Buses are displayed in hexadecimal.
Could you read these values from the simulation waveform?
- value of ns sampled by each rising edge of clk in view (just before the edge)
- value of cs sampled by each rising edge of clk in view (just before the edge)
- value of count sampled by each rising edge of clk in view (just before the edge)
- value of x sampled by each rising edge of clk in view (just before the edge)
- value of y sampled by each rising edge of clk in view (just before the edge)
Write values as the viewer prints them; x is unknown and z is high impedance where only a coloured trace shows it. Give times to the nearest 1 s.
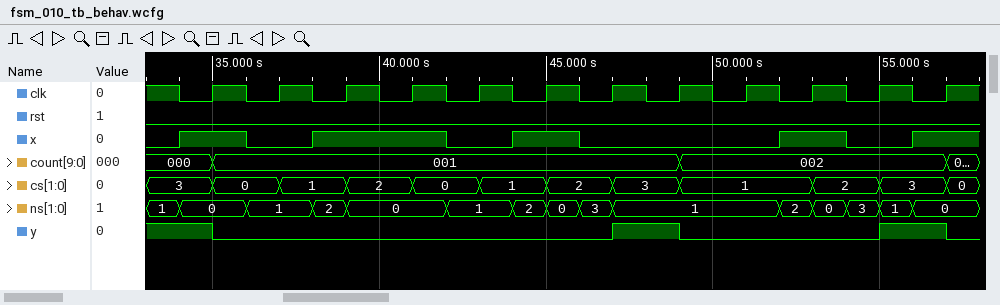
0, 1, 2, 0, 1, 2, 3, 1, 1, 2, 3, 0
3, 0, 1, 2, 0, 1, 2, 3, 1, 1, 2, 3
000, 001, 001, 001, 001, 001, 001, 001, 002, 002, 002, 002
1 0 1 1 0 1 0 0 0 1 0 1
1 0 0 0 0 0 0 1 0 0 0 1
